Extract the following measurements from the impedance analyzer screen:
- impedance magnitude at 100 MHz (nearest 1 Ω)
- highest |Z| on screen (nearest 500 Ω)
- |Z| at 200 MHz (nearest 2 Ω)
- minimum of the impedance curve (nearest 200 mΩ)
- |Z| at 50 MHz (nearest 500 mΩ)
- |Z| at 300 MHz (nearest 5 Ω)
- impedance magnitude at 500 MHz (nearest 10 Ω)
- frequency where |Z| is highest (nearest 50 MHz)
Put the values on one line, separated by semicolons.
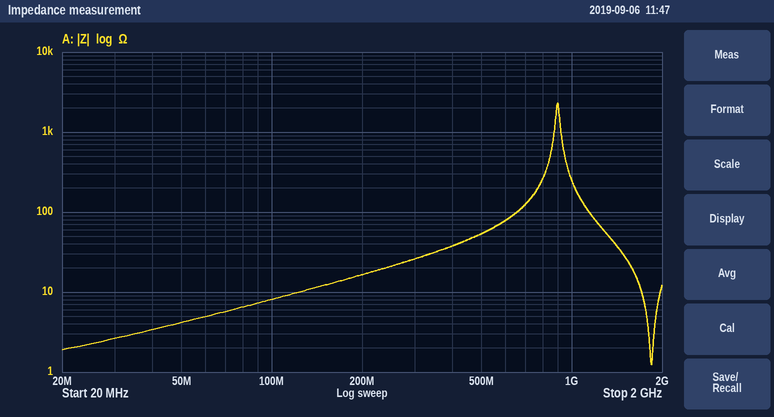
8 Ω; 2.5 kΩ; 16 Ω; 1.2 Ω; 4.0 Ω; 25 Ω; 50 Ω; 900 MHz
